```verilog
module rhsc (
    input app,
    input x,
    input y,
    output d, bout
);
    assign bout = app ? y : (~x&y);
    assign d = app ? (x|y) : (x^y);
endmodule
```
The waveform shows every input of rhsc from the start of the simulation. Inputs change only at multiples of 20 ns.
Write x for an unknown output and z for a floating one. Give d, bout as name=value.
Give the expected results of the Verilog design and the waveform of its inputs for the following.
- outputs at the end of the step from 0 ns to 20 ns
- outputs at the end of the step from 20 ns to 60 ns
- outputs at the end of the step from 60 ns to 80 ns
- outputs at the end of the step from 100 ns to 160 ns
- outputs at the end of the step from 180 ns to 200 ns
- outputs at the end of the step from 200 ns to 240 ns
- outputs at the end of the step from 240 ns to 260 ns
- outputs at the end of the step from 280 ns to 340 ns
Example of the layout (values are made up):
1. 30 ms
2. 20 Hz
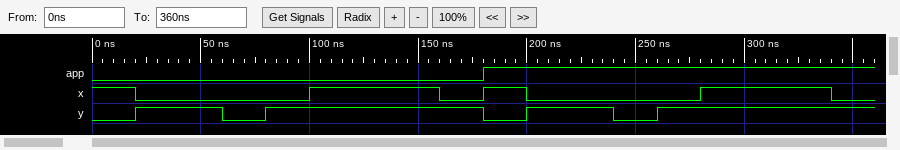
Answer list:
1. d=1, bout=0
2. d=1, bout=1
3. d=0, bout=0
4. d=0, bout=0
5. d=1, bout=0
6. d=1, bout=1
7. d=0, bout=0
8. d=1, bout=1
